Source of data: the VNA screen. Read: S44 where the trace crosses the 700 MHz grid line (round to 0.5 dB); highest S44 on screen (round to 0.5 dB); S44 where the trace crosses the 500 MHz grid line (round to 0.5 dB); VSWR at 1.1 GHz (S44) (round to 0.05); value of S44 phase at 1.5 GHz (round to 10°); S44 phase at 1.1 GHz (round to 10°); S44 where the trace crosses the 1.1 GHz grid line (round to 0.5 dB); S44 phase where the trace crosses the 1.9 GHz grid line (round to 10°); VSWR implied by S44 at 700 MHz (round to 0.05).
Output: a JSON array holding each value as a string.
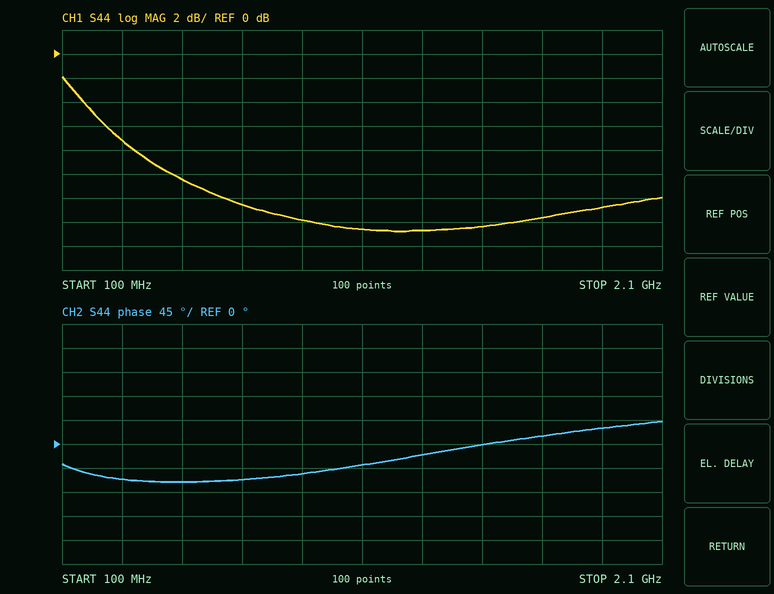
["-12.5 dB", "-2.0 dB", "-10.5 dB", "1.45", "0°", "-40°", "-14.5 dB", "30°", "1.60"]
